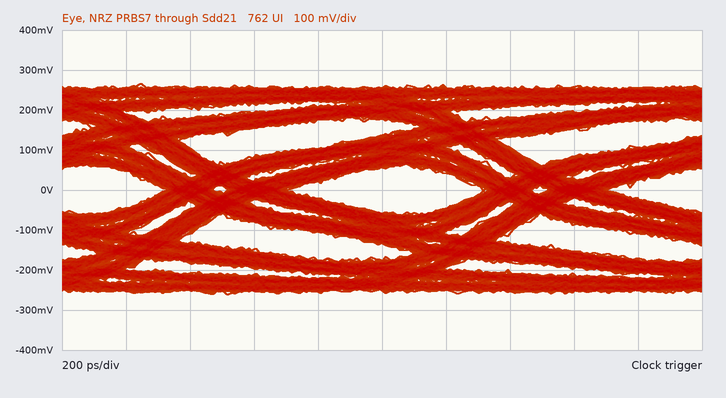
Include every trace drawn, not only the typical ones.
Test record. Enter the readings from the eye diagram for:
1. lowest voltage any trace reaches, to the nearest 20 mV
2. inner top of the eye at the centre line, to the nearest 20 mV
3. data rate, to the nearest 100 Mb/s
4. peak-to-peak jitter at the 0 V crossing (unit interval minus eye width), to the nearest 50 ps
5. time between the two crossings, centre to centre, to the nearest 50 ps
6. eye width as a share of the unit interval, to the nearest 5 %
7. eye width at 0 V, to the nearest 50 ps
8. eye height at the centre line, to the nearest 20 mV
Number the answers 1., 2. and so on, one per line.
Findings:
1. -260 mV
2. 60 mV
3. 1.0 Gb/s
4. 400 ps
5. 1.00 ns
6. 60 %
7. 600 ps
8. 120 mV
